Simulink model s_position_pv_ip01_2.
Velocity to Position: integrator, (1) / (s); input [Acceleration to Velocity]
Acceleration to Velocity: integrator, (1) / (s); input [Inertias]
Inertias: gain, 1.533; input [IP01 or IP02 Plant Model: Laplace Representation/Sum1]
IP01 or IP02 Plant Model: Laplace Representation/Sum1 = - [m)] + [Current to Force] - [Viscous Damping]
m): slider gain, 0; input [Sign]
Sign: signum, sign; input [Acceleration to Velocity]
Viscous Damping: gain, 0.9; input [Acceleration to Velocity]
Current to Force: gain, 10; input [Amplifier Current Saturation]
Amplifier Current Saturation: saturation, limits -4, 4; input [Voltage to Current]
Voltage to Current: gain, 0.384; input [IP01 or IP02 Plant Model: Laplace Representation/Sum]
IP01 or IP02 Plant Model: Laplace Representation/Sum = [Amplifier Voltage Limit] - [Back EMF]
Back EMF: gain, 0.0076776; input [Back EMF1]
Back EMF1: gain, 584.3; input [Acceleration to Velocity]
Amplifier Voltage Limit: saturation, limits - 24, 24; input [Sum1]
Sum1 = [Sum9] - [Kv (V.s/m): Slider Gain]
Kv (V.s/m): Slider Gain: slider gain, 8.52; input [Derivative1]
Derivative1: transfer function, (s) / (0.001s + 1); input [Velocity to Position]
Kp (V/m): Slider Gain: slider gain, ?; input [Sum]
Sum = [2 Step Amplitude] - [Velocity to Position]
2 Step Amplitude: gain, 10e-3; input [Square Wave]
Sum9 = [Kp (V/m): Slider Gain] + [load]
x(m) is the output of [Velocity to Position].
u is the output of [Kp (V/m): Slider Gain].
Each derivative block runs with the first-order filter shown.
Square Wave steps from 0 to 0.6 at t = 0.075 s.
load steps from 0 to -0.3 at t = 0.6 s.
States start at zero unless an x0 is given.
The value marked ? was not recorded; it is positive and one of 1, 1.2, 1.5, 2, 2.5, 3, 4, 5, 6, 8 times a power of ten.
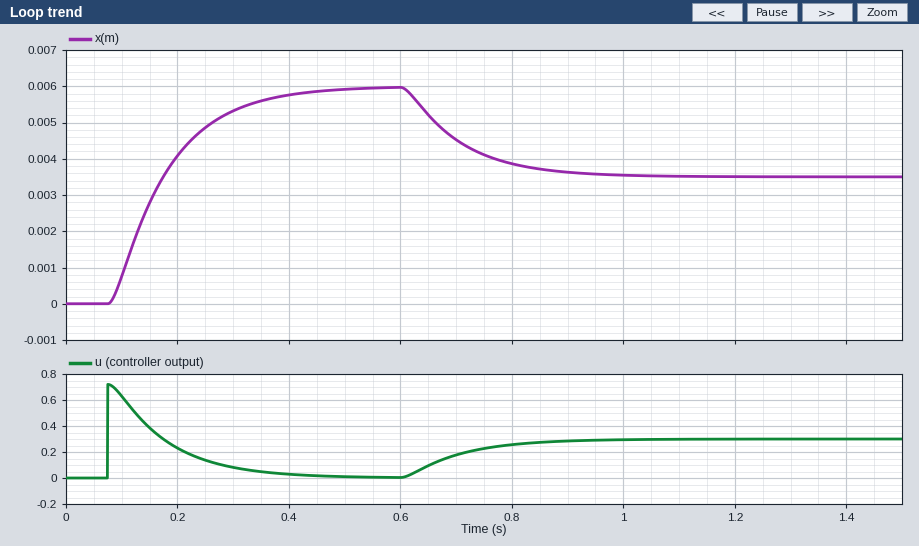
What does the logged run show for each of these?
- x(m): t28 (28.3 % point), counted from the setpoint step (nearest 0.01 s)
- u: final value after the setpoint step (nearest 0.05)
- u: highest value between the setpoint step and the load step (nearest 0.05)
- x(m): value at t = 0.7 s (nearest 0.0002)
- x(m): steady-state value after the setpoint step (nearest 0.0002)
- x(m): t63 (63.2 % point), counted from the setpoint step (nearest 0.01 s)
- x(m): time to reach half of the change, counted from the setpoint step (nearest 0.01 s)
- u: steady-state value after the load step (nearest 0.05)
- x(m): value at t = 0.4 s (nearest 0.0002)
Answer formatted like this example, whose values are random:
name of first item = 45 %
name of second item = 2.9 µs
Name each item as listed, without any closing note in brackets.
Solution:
x(m): t28 (28.3 % point), counted from the setpoint step = 0.05 s
u: final value after the setpoint step = 0.00
u: highest value between the setpoint step and the load step = 0.70
x(m): value at t = 0.7 s = 0.0046
x(m): steady-state value after the setpoint step = 0.0060
x(m): t63 (63.2 % point), counted from the setpoint step = 0.11 s
x(m): time to reach half of the change, counted from the setpoint step = 0.08 s
u: steady-state value after the load step = 0.30
x(m): value at t = 0.4 s = 0.0058
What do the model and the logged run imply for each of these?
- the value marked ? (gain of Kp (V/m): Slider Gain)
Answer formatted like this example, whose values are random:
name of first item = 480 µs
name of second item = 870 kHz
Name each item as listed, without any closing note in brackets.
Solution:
the value marked ? (gain of Kp (V/m): Slider Gain) = 120
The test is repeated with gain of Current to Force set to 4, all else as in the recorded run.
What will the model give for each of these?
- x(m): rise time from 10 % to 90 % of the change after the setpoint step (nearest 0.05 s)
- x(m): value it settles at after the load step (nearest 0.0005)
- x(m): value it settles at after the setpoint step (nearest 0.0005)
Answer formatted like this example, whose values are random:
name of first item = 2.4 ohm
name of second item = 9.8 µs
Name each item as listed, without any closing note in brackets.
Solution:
x(m): rise time from 10 % to 90 % of the change after the setpoint step = 0.20 s
x(m): value it settles at after the load step = 0.0035
x(m): value it settles at after the setpoint step = 0.0060
